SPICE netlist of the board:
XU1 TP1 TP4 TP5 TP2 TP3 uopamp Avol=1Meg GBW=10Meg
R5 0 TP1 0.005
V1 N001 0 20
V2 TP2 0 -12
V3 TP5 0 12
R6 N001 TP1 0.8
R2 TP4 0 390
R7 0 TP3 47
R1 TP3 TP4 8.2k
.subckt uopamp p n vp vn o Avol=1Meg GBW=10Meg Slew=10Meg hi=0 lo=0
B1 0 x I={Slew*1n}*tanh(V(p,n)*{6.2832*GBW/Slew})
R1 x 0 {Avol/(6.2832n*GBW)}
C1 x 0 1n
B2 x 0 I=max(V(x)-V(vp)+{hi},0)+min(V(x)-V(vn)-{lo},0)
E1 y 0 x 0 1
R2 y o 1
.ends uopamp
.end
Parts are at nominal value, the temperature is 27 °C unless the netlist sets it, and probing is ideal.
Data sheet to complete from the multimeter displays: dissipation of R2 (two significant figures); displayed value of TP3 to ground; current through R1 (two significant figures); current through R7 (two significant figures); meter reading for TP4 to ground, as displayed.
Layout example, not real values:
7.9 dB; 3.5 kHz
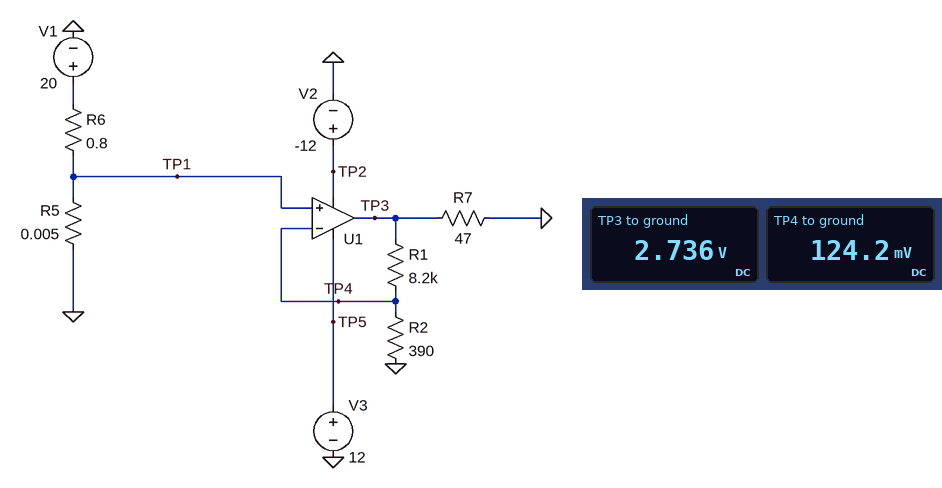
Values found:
40 µW; 2.736 V; 320 µA; 58 mA; 124.2 mV
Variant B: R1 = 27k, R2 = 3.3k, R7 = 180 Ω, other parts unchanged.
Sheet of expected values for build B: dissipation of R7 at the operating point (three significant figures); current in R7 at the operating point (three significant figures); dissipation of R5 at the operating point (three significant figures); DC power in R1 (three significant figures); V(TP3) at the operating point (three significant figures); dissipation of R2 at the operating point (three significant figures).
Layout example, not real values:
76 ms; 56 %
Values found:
7.23 mW; 6.34 mA; 3.09 W; 38.3 µW; 1.14 V; 4.68 µW
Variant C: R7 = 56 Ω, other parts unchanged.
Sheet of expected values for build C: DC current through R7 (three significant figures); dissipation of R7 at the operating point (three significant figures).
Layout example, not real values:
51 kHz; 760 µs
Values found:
48.9 mA; 134 mW
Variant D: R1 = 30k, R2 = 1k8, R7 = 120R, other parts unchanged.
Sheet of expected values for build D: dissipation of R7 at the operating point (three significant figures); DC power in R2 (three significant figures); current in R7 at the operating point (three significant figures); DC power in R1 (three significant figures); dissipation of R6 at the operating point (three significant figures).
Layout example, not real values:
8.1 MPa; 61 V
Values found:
40.1 mW; 8.57 µW; 18.3 mA; 143 µW; 494 W
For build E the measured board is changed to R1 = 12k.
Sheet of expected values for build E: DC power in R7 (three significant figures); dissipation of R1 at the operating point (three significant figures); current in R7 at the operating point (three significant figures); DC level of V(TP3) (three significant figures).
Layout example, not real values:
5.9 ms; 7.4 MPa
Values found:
331 mW; 1.22 mW; 84.0 mA; 3.95 V
